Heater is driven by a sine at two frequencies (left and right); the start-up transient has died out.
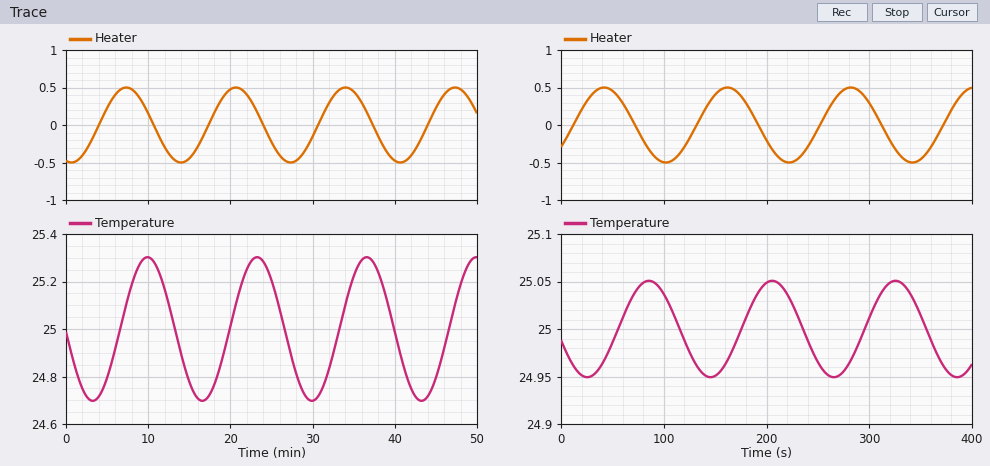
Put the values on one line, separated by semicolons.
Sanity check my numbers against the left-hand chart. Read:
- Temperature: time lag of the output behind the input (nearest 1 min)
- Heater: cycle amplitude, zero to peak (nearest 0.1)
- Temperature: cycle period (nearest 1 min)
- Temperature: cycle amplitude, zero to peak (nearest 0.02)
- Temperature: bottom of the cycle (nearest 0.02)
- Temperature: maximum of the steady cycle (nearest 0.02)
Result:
3 min; 0.5; 13 min; 0.30; 24.70; 25.30
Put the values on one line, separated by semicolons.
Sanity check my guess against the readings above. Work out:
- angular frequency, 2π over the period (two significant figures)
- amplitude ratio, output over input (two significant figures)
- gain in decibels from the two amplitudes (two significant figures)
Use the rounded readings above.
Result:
0.48 rad/min; 0.60; -4.4 dB
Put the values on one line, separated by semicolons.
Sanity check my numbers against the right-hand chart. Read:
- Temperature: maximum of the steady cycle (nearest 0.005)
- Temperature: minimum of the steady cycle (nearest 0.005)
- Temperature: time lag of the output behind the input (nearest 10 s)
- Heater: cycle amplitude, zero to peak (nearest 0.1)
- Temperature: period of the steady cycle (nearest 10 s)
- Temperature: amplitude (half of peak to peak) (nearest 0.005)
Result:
25.050; 24.950; 40 s; 0.5; 120 s; 0.050
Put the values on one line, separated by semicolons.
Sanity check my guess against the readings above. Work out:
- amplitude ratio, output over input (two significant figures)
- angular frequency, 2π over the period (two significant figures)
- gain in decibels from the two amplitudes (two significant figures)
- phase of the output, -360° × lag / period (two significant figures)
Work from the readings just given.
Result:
0.10; 0.052 rad/s; -20 dB; -120°
